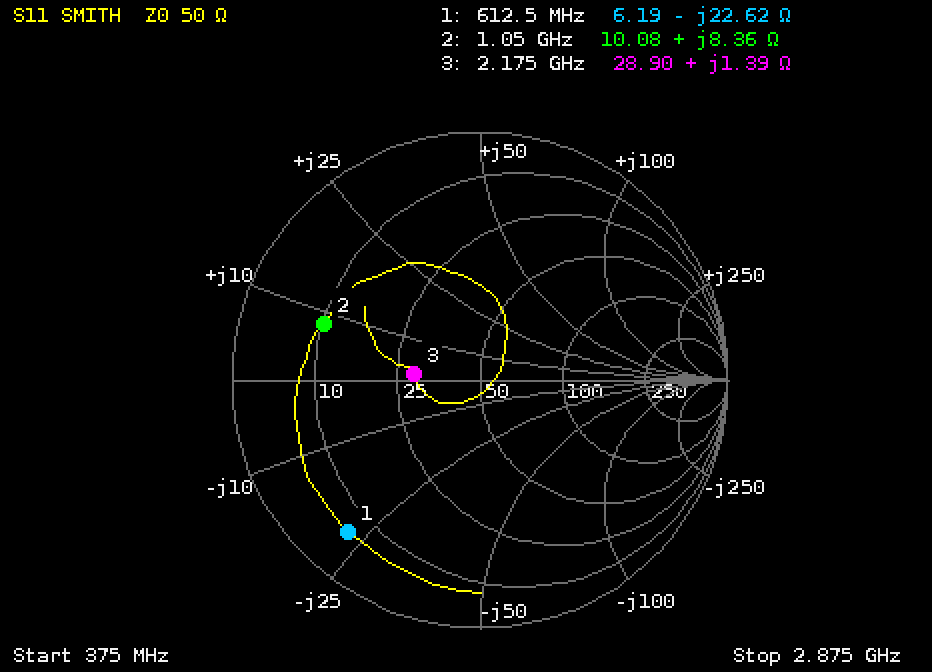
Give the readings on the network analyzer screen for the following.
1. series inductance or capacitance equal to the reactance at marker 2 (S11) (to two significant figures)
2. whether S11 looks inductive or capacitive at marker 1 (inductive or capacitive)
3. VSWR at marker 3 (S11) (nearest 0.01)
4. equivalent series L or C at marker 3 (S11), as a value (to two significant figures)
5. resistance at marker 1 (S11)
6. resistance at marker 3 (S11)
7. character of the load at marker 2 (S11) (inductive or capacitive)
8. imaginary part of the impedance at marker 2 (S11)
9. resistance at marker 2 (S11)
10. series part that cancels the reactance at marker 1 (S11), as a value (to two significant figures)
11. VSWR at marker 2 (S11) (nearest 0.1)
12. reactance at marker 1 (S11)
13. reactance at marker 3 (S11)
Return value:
1.3 nH
capacitive
1.73
100 pH
6.19 Ω
28.90 Ω
inductive
+8.36 Ω
10.08 Ω
5.9 nH
5.1
-22.62 Ω
+1.39 Ω
